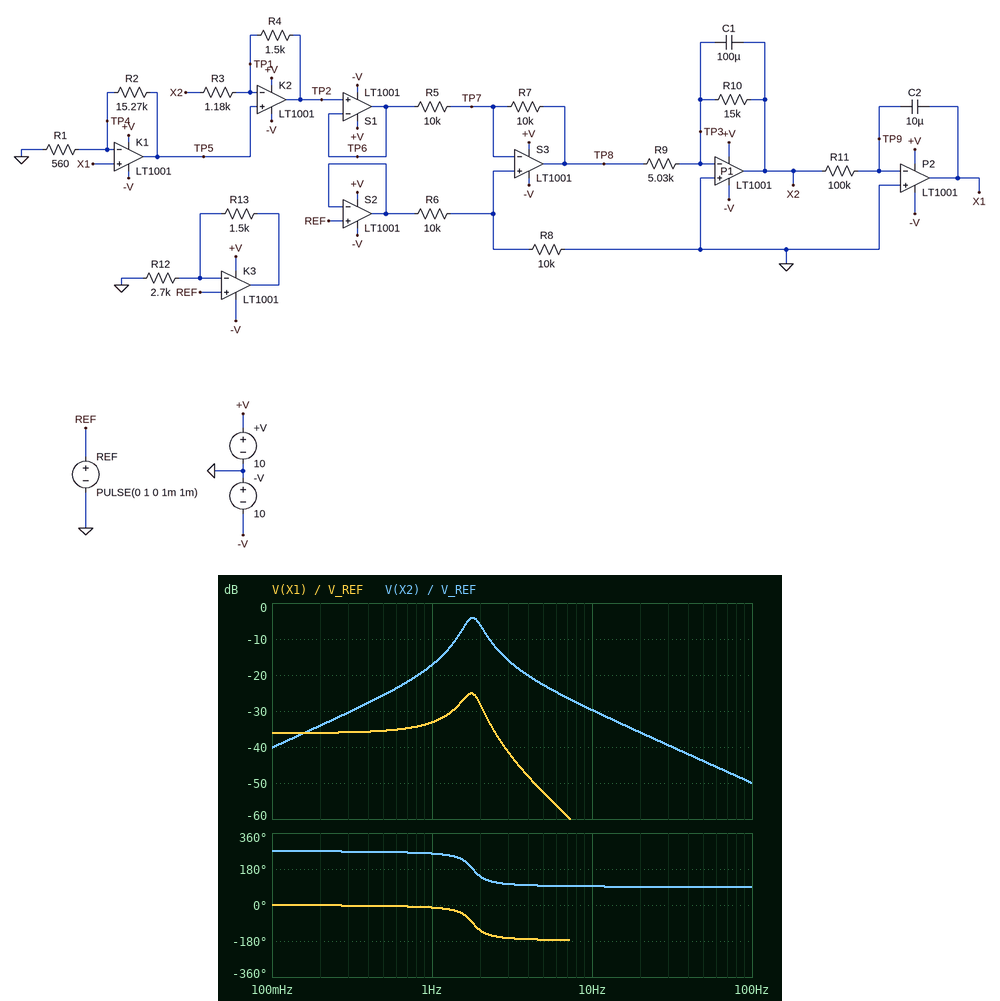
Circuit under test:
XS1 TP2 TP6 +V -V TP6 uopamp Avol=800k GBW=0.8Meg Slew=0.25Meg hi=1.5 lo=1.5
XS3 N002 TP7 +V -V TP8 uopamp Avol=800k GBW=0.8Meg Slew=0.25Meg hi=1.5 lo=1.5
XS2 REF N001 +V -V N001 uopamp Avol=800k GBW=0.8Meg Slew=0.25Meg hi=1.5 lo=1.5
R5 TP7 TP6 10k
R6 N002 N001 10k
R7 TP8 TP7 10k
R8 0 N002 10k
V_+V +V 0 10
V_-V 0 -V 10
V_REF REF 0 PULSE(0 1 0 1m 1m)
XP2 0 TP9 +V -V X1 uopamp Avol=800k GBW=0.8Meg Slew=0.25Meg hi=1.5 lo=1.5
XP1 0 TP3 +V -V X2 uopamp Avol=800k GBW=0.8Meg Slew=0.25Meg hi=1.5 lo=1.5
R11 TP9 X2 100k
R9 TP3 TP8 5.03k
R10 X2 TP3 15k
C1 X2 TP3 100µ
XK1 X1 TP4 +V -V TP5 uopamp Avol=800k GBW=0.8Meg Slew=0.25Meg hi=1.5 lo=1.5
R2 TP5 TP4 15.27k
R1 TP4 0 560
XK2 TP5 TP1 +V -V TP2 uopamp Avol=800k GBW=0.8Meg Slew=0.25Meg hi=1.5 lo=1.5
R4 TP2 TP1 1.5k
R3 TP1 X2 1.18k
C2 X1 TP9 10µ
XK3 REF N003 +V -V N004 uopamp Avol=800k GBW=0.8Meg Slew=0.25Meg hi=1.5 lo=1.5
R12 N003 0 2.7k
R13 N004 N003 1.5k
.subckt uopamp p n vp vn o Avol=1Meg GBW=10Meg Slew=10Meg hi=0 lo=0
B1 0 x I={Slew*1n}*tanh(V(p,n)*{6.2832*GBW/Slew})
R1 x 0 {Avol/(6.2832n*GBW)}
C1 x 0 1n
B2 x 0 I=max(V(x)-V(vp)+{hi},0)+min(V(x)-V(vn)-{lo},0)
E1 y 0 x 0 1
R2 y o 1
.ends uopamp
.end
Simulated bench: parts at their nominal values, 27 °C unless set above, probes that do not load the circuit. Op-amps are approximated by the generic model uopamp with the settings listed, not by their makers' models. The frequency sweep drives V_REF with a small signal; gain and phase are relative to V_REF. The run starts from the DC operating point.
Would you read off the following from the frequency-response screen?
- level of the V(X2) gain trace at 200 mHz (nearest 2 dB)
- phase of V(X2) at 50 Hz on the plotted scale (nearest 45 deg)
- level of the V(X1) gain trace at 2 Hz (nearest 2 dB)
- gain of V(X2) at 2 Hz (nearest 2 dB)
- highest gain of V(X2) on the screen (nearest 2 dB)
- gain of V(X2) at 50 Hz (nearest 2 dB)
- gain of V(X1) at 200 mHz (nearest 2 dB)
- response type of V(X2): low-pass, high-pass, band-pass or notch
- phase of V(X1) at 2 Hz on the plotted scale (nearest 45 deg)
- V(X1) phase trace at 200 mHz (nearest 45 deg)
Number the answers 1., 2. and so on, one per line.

1. -34 dB
2. 90 deg
3. -28 dB
4. -6 dB
5. -4 dB
6. -44 dB
7. -36 dB
8. band-pass
9. -135 deg
10. 0 deg
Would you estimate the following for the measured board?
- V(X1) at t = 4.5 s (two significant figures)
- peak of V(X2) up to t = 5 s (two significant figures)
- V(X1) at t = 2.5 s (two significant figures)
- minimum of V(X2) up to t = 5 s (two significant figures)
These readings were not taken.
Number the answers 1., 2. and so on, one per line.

1. 16 mV
2. 92 mV
3. 16 mV
4. -140 mV
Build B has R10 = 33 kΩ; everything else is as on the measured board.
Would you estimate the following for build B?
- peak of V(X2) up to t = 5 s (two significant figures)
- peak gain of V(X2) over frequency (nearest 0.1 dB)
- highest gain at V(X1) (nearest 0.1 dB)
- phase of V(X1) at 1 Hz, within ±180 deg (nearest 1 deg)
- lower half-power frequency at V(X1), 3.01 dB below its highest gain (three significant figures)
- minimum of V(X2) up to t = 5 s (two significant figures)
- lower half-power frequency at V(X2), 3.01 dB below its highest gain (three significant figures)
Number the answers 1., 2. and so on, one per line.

1. 99 mV
2. -3.1 dB
3. -24.1 dB
4. -11 deg
5. 1.53 Hz
6. -150 mV
7. 1.59 Hz
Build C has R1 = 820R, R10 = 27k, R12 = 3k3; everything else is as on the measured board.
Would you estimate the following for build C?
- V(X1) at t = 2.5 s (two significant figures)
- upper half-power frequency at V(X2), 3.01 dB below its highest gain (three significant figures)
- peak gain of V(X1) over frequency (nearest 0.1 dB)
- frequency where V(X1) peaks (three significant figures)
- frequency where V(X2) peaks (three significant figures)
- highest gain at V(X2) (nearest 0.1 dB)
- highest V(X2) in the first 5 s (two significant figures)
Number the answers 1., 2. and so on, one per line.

1. 23 mV
2. 1.75 Hz
3. -22.6 dB
4. 1.46 Hz
5. 1.50 Hz
6. -3.3 dB
7. 100 mV
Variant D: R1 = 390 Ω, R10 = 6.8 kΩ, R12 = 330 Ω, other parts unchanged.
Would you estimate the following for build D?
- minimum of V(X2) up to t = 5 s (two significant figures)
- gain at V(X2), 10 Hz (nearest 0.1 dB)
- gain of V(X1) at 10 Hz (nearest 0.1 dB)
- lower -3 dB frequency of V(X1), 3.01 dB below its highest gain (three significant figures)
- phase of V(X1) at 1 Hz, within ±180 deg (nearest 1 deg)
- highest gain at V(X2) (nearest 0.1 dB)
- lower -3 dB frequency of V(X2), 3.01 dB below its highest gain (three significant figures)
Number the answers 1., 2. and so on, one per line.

1. -120 mV
2. -29.6 dB
3. -65.6 dB
4. 1.74 Hz
5. -10 deg
6. -6.1 dB
7. 1.85 Hz
